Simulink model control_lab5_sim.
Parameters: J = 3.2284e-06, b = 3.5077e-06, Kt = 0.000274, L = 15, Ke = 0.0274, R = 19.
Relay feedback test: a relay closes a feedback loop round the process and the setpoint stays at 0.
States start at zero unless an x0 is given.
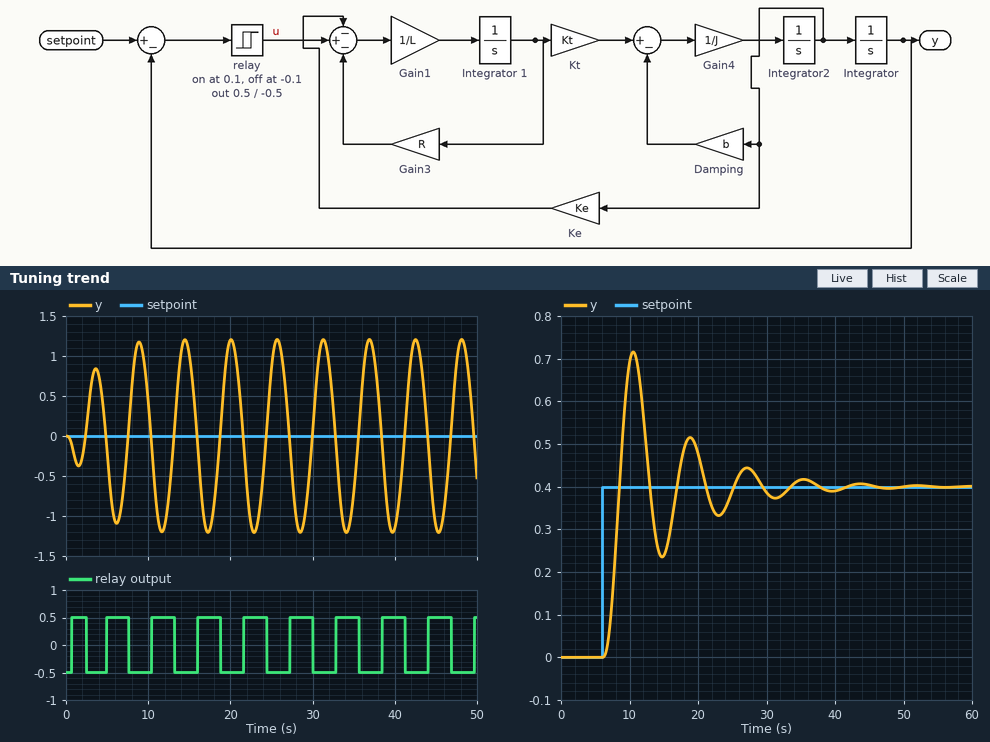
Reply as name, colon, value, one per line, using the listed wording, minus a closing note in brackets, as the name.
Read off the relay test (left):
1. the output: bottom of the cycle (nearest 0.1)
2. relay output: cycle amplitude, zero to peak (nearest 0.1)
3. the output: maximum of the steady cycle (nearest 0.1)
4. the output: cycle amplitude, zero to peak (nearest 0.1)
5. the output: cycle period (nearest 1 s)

the output: bottom of the cycle: -1.2
relay output: cycle amplitude, zero to peak: 0.5
the output: maximum of the steady cycle: 1.2
the output: cycle amplitude, zero to peak: 1.2
the output: cycle period: 6 s
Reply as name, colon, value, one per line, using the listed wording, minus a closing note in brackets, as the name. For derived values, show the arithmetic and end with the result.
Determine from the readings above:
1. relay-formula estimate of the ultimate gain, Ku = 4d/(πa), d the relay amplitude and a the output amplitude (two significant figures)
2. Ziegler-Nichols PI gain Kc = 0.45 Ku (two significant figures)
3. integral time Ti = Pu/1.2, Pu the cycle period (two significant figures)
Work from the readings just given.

relay-formula estimate of the ultimate gain, Ku = 4d/(πa), d the relay amplitude and a the output amplitude: 4 × 0.5 / (π × 1.2) = 0.53
Ziegler-Nichols PI gain Kc = 0.45 Ku: 0.45 × 0.53 = 0.24
integral time Ti = Pu/1.2, Pu the cycle period: 6 / 1.2 = 5.0 s
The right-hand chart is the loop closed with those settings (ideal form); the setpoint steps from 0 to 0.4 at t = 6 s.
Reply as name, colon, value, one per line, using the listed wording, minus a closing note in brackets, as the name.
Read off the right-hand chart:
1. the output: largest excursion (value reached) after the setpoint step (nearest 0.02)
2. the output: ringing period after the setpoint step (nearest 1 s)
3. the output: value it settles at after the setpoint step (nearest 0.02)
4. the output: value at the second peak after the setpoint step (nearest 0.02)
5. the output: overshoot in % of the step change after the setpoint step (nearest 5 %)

the output: largest excursion (value reached) after the setpoint step: 0.72
the output: ringing period after the setpoint step: 8 s
the output: value it settles at after the setpoint step: 0.40
the output: value at the second peak after the setpoint step: 0.52
the output: overshoot in % of the step change after the setpoint step: 80 %
